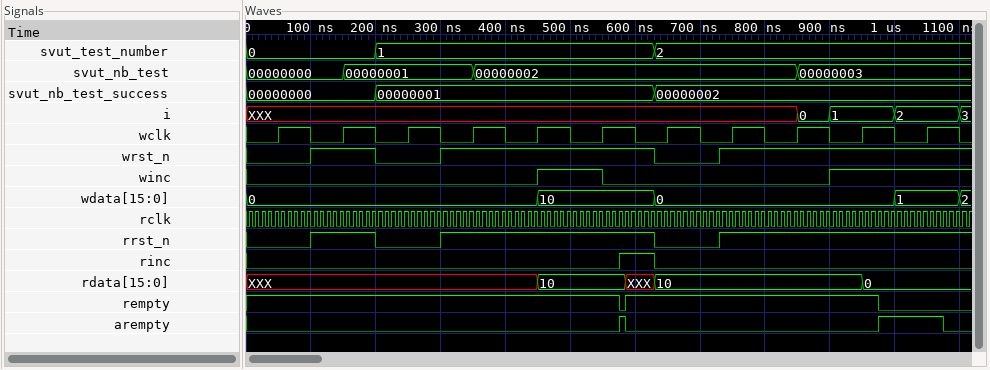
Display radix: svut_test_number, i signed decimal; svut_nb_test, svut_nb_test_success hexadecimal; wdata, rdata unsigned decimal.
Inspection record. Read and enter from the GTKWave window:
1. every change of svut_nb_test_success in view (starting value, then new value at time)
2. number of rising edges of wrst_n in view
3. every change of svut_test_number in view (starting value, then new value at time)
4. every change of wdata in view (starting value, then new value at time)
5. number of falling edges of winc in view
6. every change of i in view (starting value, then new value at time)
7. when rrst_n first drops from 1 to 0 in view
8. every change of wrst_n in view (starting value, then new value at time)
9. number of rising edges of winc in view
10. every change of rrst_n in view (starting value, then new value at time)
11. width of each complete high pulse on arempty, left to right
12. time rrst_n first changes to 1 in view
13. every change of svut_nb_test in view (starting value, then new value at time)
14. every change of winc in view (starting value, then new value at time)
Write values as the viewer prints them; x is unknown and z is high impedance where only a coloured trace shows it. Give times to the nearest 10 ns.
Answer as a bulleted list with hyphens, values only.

- 00000000, 00000001 at 200 ns, 00000002 at 630 ns
- 3
- 0, 1 at 200 ns, 2 at 630 ns
- 0, 10 at 450 ns, 0 at 630 ns, 1 at 1000 ns, 2 at 1100 ns
- 1
- XXX, 0 at 850 ns, 1 at 900 ns, 2 at 1000 ns, 3 at 1100 ns
- 200 ns
- 0, 1 at 100 ns, 0 at 200 ns, 1 at 300 ns, 0 at 630 ns, 1 at 730 ns
- 2
- 0, 1 at 100 ns, 0 at 200 ns, 1 at 300 ns, 0 at 630 ns, 1 at 730 ns
- 10 ns, 100 ns
- 100 ns
- 00000000, 00000001 at 150 ns, 00000002 at 350 ns, 00000003 at 850 ns
- 0, 1 at 450 ns, 0 at 550 ns, 1 at 900 ns
